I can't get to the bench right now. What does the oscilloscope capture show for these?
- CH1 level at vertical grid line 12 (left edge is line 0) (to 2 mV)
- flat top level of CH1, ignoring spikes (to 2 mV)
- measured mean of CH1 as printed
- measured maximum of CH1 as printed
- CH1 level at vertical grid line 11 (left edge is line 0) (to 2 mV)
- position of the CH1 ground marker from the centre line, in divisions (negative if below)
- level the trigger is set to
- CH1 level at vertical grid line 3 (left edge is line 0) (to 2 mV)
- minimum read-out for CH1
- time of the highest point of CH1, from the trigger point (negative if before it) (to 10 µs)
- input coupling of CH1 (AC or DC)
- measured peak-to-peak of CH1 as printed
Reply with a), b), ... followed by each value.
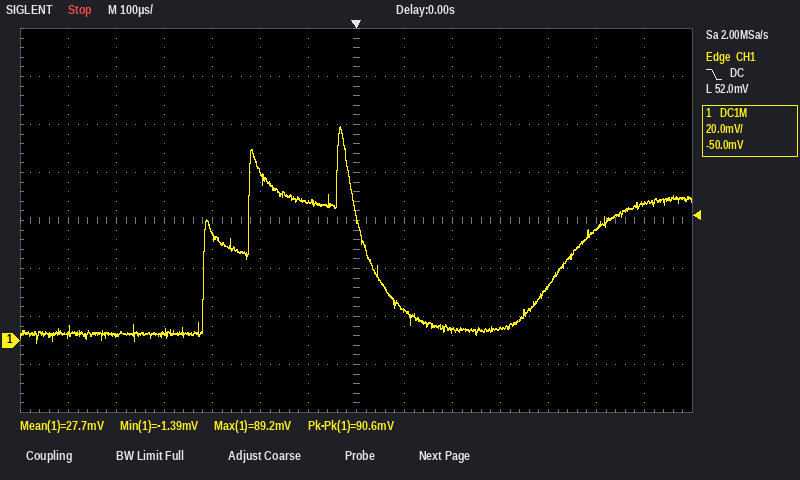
a) 46 mV
b) 58 mV
c) 27.7 mV
d) 89.2 mV
e) 22 mV
f) -2.5 div
g) 52.0 mV
h) 4 mV
i) -1.39 mV
j) -30 µs
k) DC
l) 90.6 mV
